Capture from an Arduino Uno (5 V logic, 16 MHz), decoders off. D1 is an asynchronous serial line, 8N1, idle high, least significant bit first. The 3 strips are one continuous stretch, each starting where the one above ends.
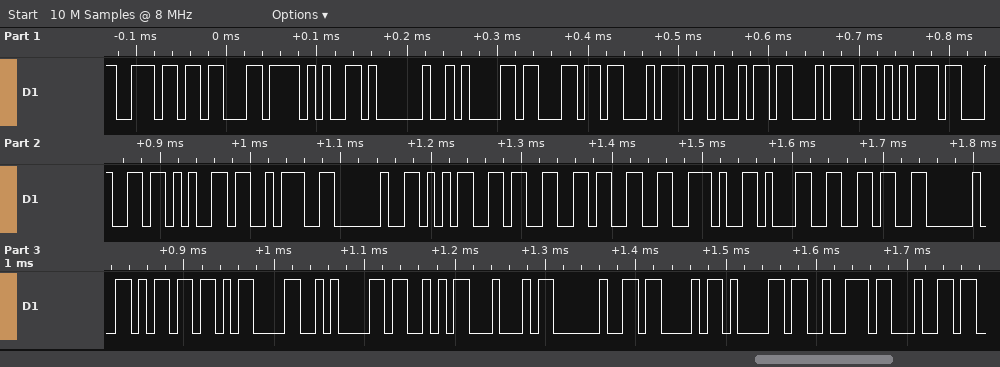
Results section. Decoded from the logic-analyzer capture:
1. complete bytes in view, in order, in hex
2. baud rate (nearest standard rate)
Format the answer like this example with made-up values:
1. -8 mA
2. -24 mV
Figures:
1. 6E 63 65 20 61 6C 74 69 74 75 64 65 3A 20 35 33 33 2E 31 36 20 6D 0D 0A 53 44 20 43 61 72 64
2. 115200 baud
